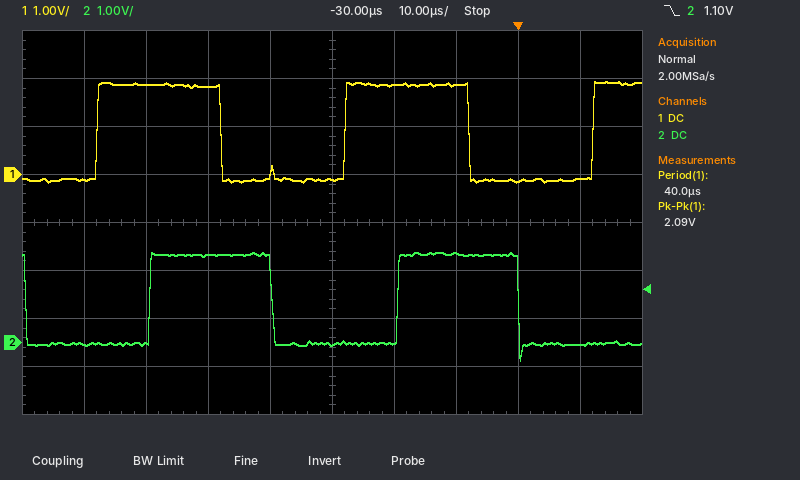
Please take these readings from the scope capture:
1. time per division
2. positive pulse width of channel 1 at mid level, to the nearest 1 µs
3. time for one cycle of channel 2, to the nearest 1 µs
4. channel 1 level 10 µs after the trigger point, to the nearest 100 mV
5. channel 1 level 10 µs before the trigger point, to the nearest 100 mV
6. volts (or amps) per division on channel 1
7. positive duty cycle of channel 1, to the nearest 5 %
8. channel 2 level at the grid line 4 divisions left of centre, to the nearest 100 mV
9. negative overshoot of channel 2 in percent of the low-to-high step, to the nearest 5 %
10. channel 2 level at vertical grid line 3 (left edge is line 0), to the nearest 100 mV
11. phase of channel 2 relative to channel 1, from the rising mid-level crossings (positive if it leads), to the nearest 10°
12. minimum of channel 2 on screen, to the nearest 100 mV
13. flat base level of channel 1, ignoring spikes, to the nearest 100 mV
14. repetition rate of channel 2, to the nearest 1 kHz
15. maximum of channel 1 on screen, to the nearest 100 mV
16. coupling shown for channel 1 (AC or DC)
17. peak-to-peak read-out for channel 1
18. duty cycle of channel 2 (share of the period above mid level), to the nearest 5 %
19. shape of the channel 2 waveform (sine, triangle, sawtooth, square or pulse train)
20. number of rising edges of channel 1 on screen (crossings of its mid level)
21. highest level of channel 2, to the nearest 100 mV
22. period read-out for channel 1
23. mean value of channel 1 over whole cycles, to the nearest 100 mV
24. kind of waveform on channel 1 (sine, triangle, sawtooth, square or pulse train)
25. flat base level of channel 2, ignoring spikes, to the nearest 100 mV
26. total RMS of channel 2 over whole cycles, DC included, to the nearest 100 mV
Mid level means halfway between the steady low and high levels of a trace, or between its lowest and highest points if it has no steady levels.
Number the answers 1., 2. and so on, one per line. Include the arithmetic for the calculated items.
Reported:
1. 10 µs
2. 20 µs
3. 40 µs
4. -100 mV
5. 1.9 V
6. 1 V
7. 50 %
8. 0.0 V
9. 20 %
10. 1.8 V
11. -80°
12. -400 mV
13. -100 mV
14. 1 / 40 µs ≈ 25 kHz
15. 1.9 V
16. DC
17. 2.09 V
18. 50 %
19. square
20. 3
21. 1.9 V
22. 40.0 µs
23. -100 mV + 0.5 × (1.9 V − (-100 mV)) ≈ 900 mV
24. square
25. 0.0 V
26. √(0.5 × (1.9 V)² + 0.5 × (0.0 V)²) ≈ 1.3 V
